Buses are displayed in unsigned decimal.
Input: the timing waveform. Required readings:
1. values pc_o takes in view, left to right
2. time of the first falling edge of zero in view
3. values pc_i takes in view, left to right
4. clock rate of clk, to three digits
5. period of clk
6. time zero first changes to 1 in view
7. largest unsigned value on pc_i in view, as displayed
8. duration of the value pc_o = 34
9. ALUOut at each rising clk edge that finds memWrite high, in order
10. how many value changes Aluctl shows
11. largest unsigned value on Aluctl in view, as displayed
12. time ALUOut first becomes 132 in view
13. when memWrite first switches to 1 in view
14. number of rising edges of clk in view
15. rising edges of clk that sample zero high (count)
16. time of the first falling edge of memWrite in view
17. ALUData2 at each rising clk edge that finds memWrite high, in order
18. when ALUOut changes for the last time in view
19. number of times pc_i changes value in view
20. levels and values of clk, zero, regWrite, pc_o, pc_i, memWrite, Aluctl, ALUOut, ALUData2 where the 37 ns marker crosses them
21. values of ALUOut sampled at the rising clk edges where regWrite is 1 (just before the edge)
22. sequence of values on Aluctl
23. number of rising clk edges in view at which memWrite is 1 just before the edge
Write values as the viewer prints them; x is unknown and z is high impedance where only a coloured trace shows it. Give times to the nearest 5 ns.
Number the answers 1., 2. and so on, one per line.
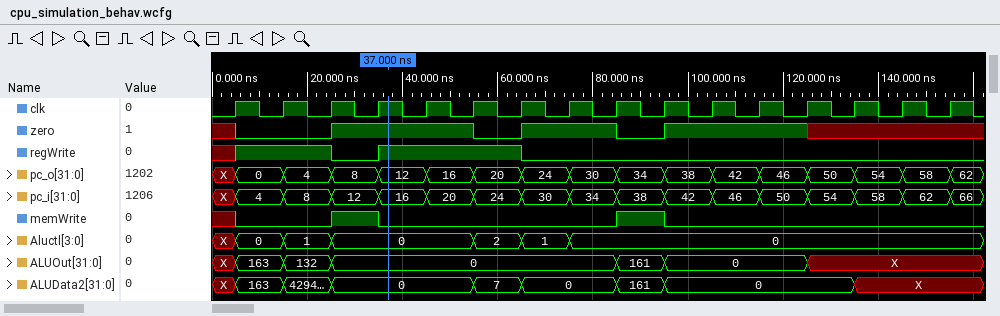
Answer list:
1. X, 0, 4, 8, 12, 16, 20, 24, 30, 34, 38, 42, 46, 50, 54, 58, 62
2. 55 ns
3. X, 4, 8, 12, 16, 20, 24, 30, 34, 38, 42, 46, 50, 54, 58, 62, 66
4. 100 MHz
5. 10 ns
6. 25 ns
7. 66
8. 10 ns
9. 0, 161
10. 6
11. 2
12. 15 ns
13. 25 ns
14. 16
15. 8
16. 35 ns
17. 0, 161
18. 125 ns
19. 16
20. clk=1, zero=1, regWrite=1, pc_o=12, pc_i=16, memWrite=0, Aluctl=0, ALUOut=0, ALUData2=0
21. 163, 132, 0, 0, 0
22. X, 0, 1, 0, 2, 1, 0
23. 2
